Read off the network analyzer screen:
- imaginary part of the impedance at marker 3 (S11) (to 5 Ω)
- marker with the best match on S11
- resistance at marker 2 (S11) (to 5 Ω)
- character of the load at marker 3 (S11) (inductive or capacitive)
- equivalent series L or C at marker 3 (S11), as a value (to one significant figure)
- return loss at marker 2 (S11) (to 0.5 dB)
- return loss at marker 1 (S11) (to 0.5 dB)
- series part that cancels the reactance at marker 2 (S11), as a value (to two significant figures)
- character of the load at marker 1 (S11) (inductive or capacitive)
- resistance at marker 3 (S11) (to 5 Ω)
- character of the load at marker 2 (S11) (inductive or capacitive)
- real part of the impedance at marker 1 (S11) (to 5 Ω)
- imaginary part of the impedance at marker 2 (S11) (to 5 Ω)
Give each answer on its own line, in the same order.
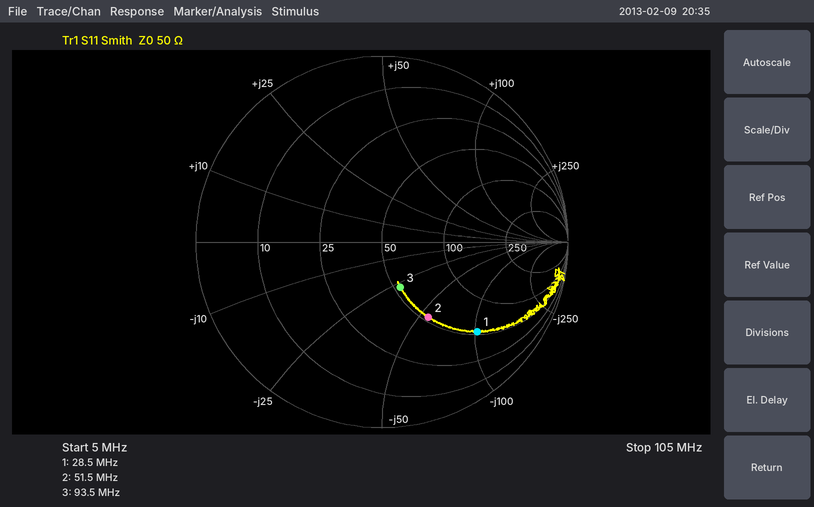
-30 Ω
marker 3
55 Ω
capacitive
60 pF
6.5 dB
3.0 dB
170 nH
capacitive
55 Ω
capacitive
55 Ω
-55 Ω
